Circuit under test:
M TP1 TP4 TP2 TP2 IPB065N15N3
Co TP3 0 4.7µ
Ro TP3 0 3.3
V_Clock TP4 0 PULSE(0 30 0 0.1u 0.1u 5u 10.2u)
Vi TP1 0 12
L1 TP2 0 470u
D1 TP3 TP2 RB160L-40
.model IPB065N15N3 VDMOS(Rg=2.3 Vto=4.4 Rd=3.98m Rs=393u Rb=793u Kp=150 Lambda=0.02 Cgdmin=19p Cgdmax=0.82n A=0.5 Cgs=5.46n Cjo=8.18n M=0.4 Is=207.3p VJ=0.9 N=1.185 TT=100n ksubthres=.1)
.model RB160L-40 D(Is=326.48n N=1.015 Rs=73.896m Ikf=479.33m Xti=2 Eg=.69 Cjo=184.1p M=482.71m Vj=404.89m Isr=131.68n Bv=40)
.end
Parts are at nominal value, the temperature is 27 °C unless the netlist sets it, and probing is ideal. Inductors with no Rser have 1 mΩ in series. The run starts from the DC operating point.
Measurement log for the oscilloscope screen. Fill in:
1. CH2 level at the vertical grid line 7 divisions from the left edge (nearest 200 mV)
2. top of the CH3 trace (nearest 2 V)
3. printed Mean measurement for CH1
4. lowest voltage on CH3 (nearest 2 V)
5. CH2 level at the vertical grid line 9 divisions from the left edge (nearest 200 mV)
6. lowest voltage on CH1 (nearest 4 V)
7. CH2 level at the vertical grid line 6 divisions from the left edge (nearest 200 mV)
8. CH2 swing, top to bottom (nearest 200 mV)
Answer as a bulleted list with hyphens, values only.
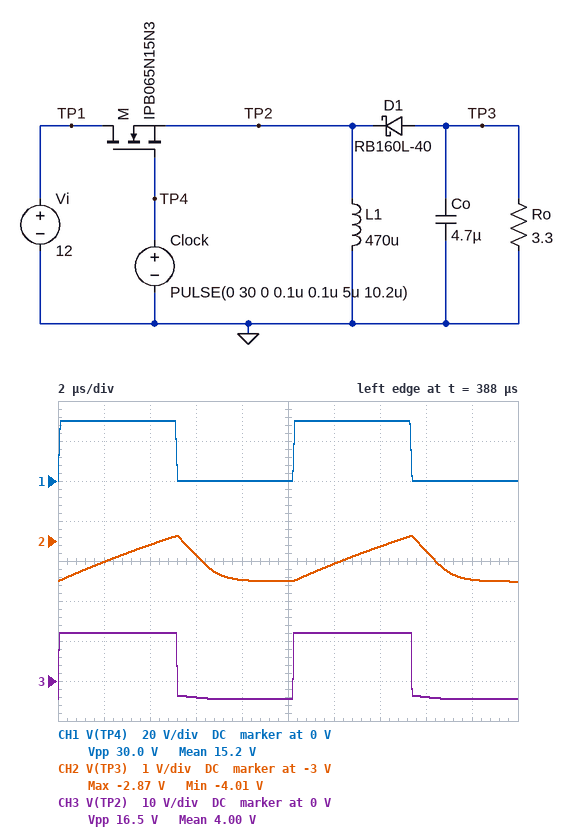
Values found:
- -3.2 V
- 12 V
- 15.2 V
- -4 V
- -4.0 V
- 0 V
- -3.6 V
- 1.2 V
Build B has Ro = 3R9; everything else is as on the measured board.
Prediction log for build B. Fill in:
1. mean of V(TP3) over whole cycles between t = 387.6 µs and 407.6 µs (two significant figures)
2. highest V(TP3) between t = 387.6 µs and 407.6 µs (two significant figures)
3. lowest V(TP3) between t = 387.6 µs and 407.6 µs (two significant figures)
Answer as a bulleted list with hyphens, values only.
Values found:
- -3.7 V
- -3.0 V
- -4.0 V
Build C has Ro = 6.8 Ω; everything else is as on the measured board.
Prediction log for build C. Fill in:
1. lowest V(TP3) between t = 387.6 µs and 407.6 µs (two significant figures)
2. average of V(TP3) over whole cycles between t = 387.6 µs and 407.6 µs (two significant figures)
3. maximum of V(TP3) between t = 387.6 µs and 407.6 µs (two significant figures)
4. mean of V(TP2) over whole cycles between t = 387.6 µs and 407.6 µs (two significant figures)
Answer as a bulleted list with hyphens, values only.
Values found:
- -4.1 V
- -3.9 V
- -3.5 V
- 3.8 V
